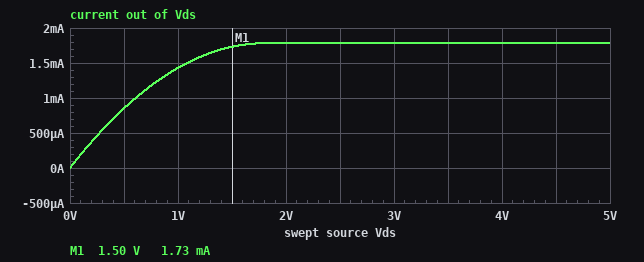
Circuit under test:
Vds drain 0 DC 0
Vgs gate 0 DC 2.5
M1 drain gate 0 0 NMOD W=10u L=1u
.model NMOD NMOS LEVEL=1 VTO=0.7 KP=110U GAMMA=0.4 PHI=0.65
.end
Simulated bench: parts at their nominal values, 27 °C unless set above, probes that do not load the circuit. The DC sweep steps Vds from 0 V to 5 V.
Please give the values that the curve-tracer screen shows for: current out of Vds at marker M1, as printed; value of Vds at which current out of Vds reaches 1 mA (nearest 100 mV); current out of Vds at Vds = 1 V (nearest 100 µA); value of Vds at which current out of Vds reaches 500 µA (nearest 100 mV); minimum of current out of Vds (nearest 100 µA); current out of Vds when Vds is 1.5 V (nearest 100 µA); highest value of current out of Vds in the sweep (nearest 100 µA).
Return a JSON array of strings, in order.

["1.73 mA", "600 mV", "1.4 mA", "300 mV", "0 A", "1.7 mA", "1.8 mA"]
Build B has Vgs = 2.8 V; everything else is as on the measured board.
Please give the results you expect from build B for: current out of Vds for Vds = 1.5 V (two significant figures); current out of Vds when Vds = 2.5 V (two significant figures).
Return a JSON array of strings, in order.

["2.2 mA", "2.4 mA"]
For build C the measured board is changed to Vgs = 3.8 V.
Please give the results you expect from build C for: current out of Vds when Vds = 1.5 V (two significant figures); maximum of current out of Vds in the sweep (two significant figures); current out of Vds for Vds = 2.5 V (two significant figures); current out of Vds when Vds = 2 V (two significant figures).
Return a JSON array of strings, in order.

["3.9 mA", "5.3 mA", "5.1 mA", "4.6 mA"]
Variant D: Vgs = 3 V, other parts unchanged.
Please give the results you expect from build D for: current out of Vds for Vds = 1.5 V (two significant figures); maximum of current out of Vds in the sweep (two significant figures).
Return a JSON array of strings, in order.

["2.6 mA", "2.9 mA"]
